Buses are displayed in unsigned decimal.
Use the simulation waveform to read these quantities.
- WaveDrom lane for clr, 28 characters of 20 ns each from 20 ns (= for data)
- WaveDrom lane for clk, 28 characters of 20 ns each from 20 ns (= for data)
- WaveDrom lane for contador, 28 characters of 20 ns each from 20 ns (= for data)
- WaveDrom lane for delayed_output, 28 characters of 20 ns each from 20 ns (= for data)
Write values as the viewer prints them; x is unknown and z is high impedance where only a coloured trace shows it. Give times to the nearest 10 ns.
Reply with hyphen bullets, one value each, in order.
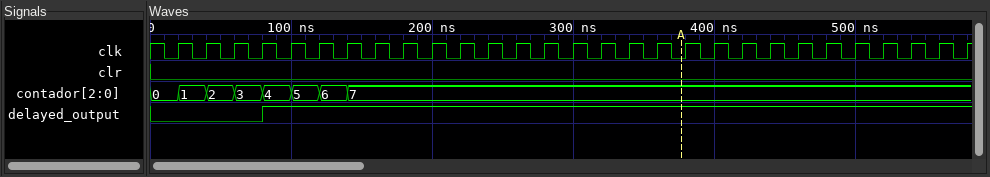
- {name: 'clr', wave: '0...........................'}
- {name: 'clk', wave: 'p...........................'}
- {name: 'contador', wave: '=======.....................', data: '1 2 3 4 5 6 7'}
- {name: 'delayed_output', wave: '0..1........................'}
